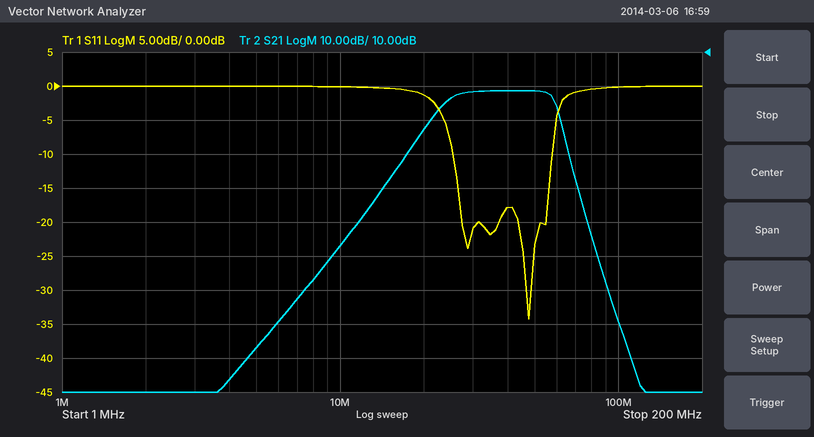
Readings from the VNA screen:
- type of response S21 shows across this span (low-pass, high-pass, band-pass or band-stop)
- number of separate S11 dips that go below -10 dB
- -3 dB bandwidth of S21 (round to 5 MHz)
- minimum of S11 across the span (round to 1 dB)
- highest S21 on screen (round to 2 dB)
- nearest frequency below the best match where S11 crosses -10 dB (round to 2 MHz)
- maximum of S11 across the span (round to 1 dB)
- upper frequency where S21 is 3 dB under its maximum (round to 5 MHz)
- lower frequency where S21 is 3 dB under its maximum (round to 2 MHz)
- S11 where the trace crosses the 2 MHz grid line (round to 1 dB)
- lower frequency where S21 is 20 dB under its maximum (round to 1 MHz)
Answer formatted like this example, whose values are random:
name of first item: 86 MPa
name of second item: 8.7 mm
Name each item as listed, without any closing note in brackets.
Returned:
type of response S21 shows across this span: band-pass
number of separate S11 dips that go below -10 dB: 2
-3 dB bandwidth of S21: 35 MHz
minimum of S11 across the span: -34 dB
highest S21 on screen: -2 dB
nearest frequency below the best match where S11 crosses -10 dB: 26 MHz
maximum of S11 across the span: 0 dB
upper frequency where S21 is 3 dB under its maximum: 60 MHz
lower frequency where S21 is 3 dB under its maximum: 24 MHz
S11 where the trace crosses the 2 MHz grid line: 0 dB
lower frequency where S21 is 20 dB under its maximum: 17 MHz
